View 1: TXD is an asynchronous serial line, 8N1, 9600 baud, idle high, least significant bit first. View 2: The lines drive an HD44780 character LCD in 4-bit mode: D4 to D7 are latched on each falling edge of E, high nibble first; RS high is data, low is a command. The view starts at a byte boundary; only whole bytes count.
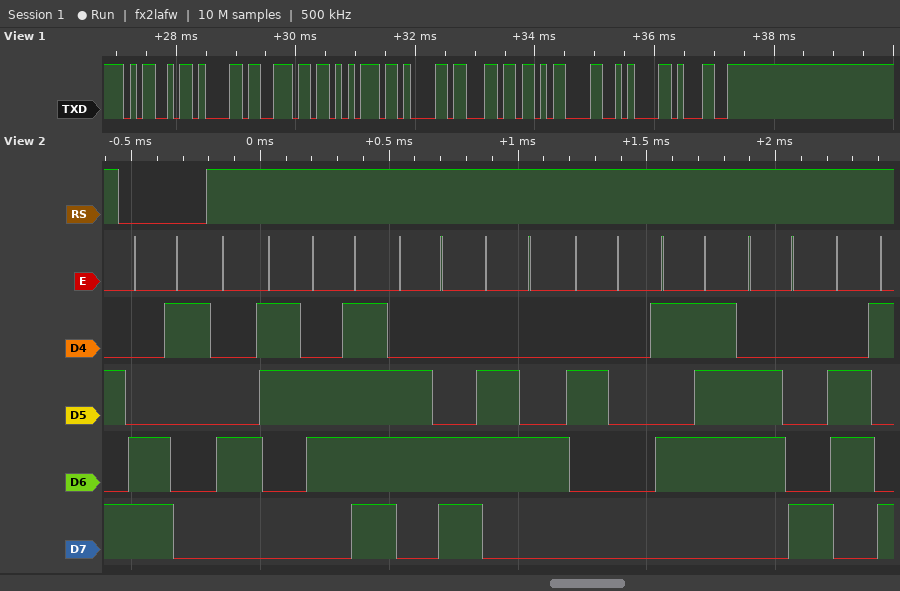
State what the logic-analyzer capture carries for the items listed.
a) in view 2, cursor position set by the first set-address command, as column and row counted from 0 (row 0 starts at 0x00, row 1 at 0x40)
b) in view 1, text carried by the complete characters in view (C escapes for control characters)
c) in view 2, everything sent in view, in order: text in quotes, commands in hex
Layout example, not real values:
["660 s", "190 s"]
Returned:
["column 1, row 1", "\"Manual\\r\\n1\"", "0xC1 \"Cold Whi\""]
